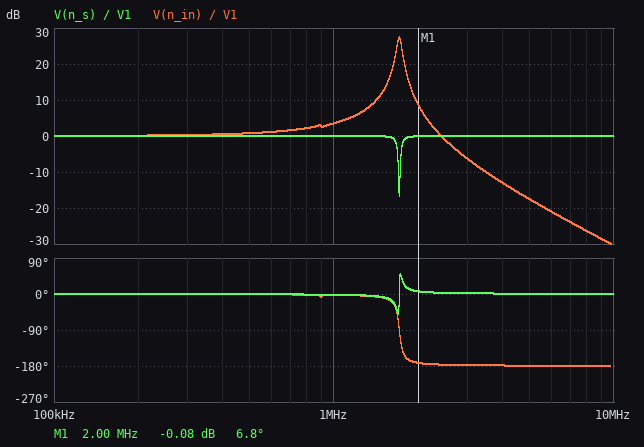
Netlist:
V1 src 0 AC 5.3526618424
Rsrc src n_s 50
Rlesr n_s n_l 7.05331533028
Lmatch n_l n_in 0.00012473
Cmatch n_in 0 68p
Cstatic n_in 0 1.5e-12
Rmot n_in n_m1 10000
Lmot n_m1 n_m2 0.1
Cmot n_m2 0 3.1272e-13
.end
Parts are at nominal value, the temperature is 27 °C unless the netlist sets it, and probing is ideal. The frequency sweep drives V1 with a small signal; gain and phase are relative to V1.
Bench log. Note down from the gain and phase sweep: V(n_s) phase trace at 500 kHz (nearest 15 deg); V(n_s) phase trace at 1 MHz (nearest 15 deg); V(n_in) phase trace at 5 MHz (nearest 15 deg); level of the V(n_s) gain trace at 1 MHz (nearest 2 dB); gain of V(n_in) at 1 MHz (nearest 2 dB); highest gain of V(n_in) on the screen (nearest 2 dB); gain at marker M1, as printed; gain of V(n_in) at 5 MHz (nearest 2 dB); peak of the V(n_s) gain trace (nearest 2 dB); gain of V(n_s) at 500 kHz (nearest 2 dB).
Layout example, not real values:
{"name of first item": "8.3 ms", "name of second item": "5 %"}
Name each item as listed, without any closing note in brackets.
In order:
{"V(n_s) phase trace at 500 kHz": "0 deg", "V(n_s) phase trace at 1 MHz": "0 deg", "V(n_in) phase trace at 5 MHz": "-180 deg", "level of the V(n_s) gain trace at 1 MHz": "0 dB", "gain of V(n_in) at 1 MHz": "4 dB", "highest gain of V(n_in) on the screen": "28 dB", "gain at marker M1, as printed": "-0.08 dB", "gain of V(n_in) at 5 MHz": "-18 dB", "peak of the V(n_s) gain trace": "0 dB", "gain of V(n_s) at 500 kHz": "0 dB"}
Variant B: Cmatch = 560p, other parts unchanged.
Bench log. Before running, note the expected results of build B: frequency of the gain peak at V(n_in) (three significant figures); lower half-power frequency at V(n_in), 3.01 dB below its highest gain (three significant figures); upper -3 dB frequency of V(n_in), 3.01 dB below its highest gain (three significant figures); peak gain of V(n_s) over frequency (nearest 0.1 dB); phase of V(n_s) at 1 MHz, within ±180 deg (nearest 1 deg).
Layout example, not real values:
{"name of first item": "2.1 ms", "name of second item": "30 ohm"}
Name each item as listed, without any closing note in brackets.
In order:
{"frequency of the gain peak at V(n_in)": "599 kHz", "lower half-power frequency at V(n_in), 3.01 dB below its highest gain": "561 kHz", "upper -3 dB frequency of V(n_in), 3.01 dB below its highest gain": "634 kHz", "peak gain of V(n_s) over frequency": "0 dB", "phase of V(n_s) at 1 MHz, within ±180 deg": "6 deg"}
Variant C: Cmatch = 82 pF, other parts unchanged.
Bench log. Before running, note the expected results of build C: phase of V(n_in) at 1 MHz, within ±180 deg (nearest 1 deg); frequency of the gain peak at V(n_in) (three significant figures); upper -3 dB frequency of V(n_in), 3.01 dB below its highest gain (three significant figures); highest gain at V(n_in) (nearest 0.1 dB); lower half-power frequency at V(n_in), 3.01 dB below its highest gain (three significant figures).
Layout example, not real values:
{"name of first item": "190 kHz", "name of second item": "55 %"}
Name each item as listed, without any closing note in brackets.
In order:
{"phase of V(n_in) at 1 MHz, within ±180 deg": "-3 deg", "frequency of the gain peak at V(n_in)": "1.56 MHz", "upper -3 dB frequency of V(n_in), 3.01 dB below its highest gain": "1.60 MHz", "highest gain at V(n_in)": "26.6 dB", "lower half-power frequency at V(n_in), 3.01 dB below its highest gain": "1.52 MHz"}
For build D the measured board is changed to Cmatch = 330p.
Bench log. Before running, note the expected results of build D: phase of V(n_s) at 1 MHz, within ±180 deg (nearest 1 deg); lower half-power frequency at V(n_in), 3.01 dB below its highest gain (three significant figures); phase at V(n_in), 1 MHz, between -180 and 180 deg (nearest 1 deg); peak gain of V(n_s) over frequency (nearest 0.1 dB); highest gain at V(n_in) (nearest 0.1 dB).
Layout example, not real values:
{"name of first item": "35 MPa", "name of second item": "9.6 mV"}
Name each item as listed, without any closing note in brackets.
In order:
{"phase of V(n_s) at 1 MHz, within ±180 deg": "9 deg", "lower half-power frequency at V(n_in), 3.01 dB below its highest gain": "742 kHz", "phase at V(n_in), 1 MHz, between -180 and 180 deg": "-169 deg", "peak gain of V(n_s) over frequency": "0 dB", "highest gain at V(n_in)": "20.6 dB"}
